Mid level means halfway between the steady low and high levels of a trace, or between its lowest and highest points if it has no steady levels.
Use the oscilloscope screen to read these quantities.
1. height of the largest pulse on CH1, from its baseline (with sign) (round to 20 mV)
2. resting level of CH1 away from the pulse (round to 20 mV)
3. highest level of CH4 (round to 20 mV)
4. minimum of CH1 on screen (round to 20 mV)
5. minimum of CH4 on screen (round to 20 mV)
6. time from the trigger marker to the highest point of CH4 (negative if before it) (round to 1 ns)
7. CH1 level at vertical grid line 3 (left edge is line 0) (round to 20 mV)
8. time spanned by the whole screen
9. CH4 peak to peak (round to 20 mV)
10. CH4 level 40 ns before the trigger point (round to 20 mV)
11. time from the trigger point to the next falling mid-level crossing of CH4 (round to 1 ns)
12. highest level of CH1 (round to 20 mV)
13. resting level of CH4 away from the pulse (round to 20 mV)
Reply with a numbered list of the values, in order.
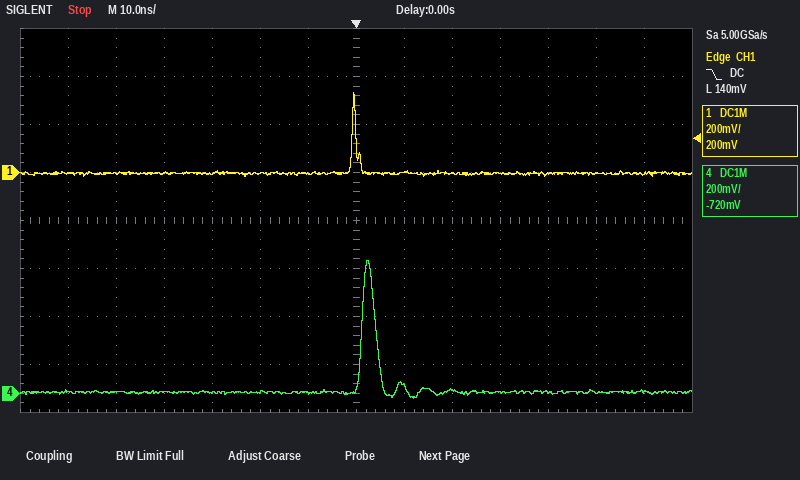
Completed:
1. +340 mV
2. 0 mV
3. 560 mV
4. -20 mV
5. -20 mV
6. +2 ns
7. 0 mV
8. 140 ns
9. 580 mV
10. 0 mV
11. 4 ns
12. 340 mV
13. 0 mV
